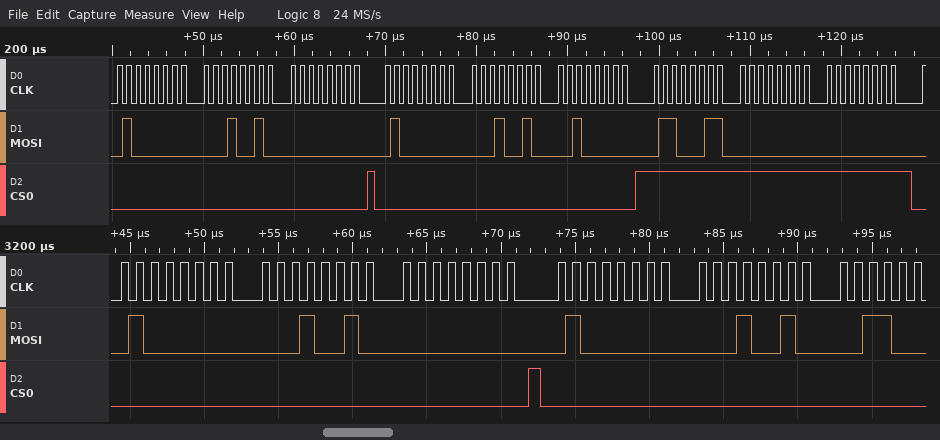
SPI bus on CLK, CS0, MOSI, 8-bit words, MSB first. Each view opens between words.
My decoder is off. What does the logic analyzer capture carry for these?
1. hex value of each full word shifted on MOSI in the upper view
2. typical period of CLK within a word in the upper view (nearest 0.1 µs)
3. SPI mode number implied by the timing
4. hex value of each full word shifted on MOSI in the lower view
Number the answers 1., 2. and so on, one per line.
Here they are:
1. 40, 12, 00, 40, 12, 20, 63, 00, 00
2. 1 µs
3. 0
4. 40, 12, 00, 40, 12
